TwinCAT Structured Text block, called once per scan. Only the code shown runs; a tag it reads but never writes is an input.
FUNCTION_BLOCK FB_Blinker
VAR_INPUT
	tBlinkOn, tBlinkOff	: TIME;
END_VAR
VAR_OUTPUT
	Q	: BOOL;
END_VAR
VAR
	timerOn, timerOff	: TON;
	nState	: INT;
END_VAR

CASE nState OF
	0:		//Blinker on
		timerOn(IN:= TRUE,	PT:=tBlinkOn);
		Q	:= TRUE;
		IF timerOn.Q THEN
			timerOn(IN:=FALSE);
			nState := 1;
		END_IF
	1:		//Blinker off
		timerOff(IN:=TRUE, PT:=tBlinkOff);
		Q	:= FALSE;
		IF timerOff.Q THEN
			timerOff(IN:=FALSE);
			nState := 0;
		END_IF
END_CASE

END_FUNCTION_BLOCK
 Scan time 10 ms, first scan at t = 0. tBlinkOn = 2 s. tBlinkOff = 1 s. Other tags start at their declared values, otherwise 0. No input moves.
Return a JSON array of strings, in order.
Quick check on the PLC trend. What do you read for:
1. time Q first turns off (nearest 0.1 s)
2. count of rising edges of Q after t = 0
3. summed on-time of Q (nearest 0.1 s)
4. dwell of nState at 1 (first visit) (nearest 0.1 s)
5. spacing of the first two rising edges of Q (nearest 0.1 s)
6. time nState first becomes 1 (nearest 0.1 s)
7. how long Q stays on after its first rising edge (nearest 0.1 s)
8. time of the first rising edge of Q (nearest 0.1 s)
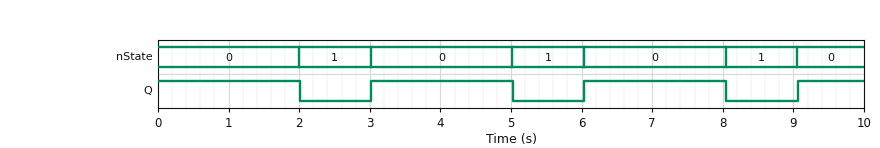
["2.0 s", "3", "7.0 s", "1.0 s", "3.0 s", "2.0 s", "2.0 s", "3.0 s"]
